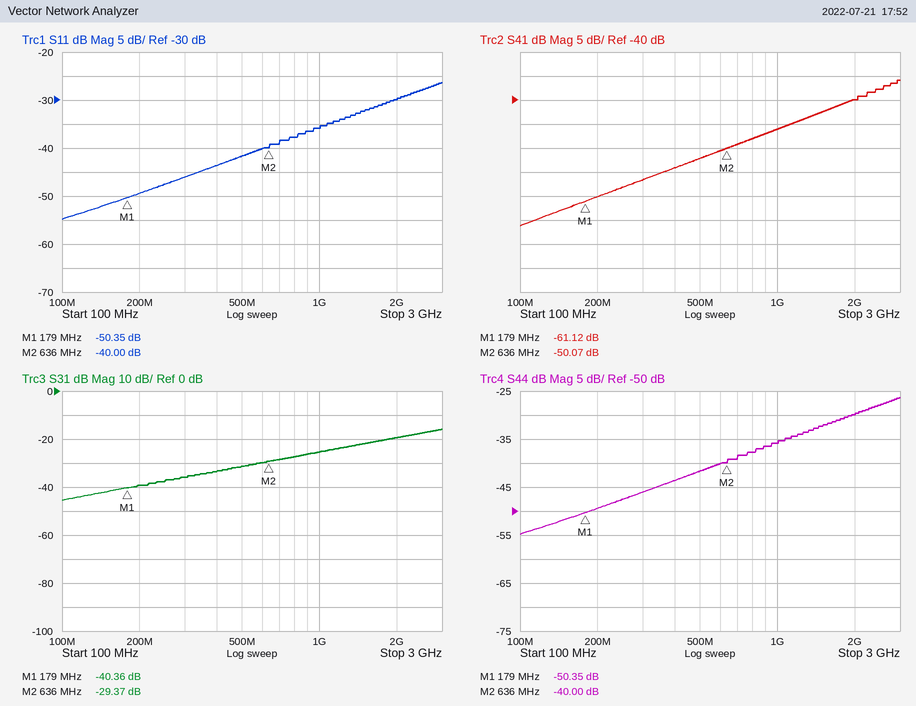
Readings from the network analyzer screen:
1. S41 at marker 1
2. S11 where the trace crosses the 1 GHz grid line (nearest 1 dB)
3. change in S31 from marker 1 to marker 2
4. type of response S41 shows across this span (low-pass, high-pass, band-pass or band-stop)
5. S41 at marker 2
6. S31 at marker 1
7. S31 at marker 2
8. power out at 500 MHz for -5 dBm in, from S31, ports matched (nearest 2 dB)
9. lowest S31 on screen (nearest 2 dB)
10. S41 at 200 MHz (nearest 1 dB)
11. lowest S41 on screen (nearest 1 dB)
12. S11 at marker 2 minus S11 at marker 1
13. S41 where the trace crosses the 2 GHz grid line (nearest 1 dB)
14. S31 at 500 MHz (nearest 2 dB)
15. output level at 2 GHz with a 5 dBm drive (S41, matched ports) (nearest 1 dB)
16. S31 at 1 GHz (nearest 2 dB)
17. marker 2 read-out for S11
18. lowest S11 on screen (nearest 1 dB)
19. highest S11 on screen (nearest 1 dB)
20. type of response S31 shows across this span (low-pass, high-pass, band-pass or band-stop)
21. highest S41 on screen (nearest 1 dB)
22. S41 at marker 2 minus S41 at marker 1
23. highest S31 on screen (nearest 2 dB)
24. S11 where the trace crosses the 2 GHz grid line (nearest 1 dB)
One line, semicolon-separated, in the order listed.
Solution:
-61.12 dB; -36 dB; 10.99 dB; high-pass; -50.07 dB; -40.36 dB; -29.37 dB; -36 dBm; -46 dB; -60 dB; -66 dB; 10.35 dB; -40 dB; -32 dB; -35 dBm; -26 dB; -40.00 dB; -55 dB; -26 dB; high-pass; -36 dB; 11.05 dB; -16 dB; -30 dB
